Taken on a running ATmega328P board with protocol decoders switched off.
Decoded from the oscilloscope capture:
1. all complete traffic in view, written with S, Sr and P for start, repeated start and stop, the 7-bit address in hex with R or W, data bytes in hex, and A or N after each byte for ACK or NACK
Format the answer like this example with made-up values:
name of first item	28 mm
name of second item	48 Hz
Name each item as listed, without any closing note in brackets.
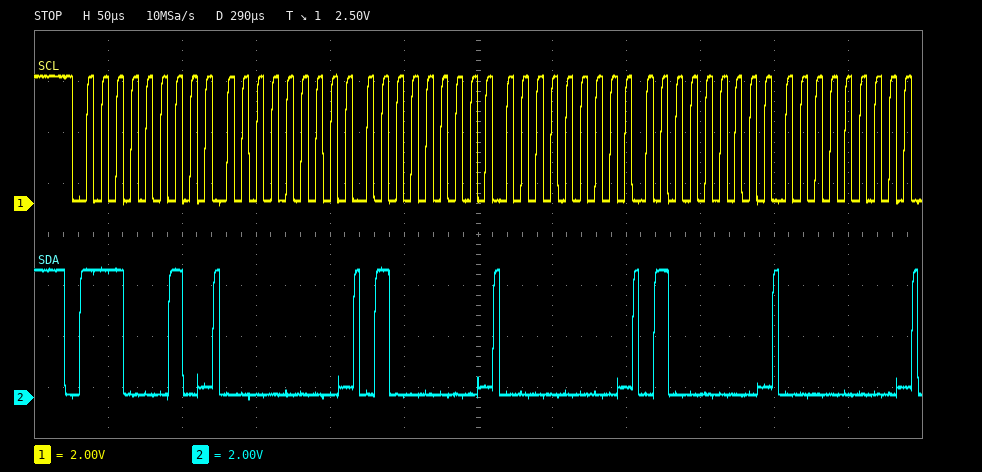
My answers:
all complete traffic in view, written with S, Sr and P for start, repeated start and stop, the 7-bit address in hex with R or W, data bytes in hex, and A or N after each byte for ACK or NACK	S 71W A 00 A 40 A 00 A 40 A 00 A
